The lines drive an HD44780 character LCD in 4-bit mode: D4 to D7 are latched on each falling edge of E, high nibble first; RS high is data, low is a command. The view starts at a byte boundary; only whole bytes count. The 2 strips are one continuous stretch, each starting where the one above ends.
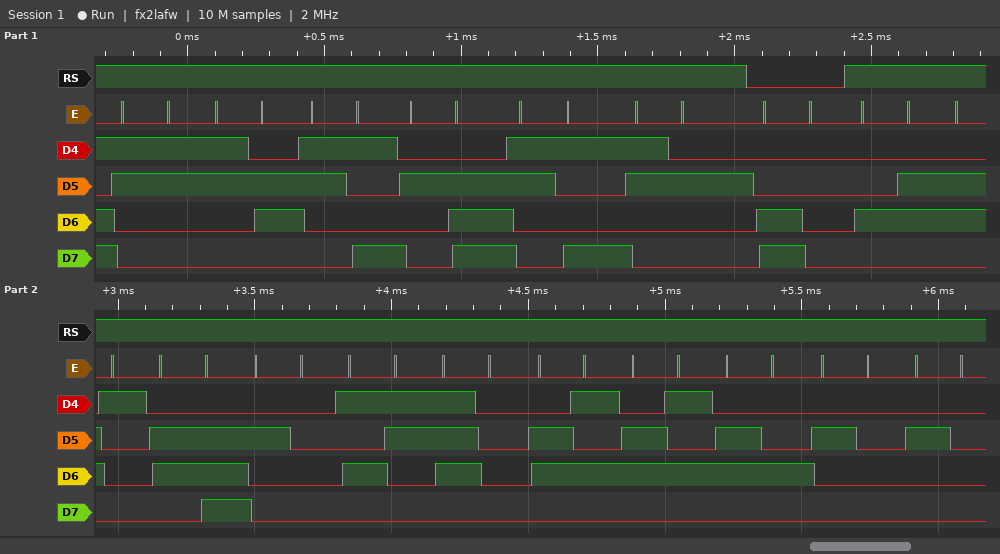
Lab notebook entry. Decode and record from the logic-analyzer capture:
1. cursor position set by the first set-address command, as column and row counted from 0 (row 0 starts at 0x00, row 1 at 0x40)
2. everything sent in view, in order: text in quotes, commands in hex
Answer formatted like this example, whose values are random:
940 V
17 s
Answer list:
column 0, row 1
"369.92" 0xC0 "Fan Speed  "
